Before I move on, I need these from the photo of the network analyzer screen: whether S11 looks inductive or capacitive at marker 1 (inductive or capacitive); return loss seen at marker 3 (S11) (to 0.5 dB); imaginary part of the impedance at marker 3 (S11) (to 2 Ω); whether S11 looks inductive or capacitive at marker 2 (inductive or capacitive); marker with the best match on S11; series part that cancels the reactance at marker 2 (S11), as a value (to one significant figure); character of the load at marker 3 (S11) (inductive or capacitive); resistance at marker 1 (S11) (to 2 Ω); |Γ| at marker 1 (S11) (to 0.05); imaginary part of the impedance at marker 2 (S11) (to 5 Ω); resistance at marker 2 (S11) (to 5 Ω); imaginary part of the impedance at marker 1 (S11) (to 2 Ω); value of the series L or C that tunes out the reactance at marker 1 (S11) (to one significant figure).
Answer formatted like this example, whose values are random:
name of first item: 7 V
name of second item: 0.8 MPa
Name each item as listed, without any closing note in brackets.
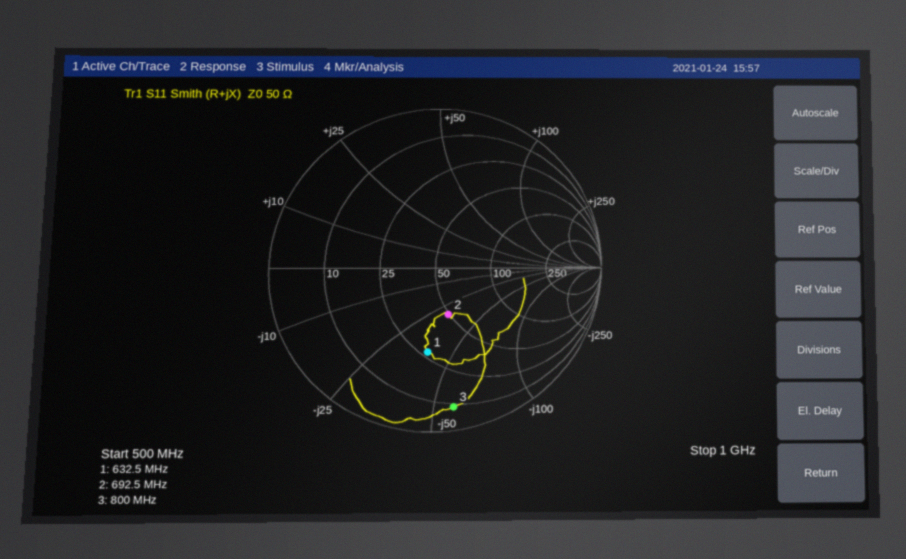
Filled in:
whether S11 looks inductive or capacitive at marker 1: capacitive
return loss seen at marker 3 (S11): 1.5 dB
imaginary part of the impedance at marker 3 (S11): -58 Ω
whether S11 looks inductive or capacitive at marker 2: capacitive
marker with the best match on S11: marker 2
series part that cancels the reactance at marker 2 (S11), as a value: 7 nH
character of the load at marker 3 (S11): capacitive
resistance at marker 1 (S11): 28 Ω
|Γ| at marker 1 (S11): 0.50
imaginary part of the impedance at marker 2 (S11): -30 Ω
resistance at marker 2 (S11): 50 Ω
imaginary part of the impedance at marker 1 (S11): -38 Ω
value of the series L or C that tunes out the reactance at marker 1 (S11): 10 nH
